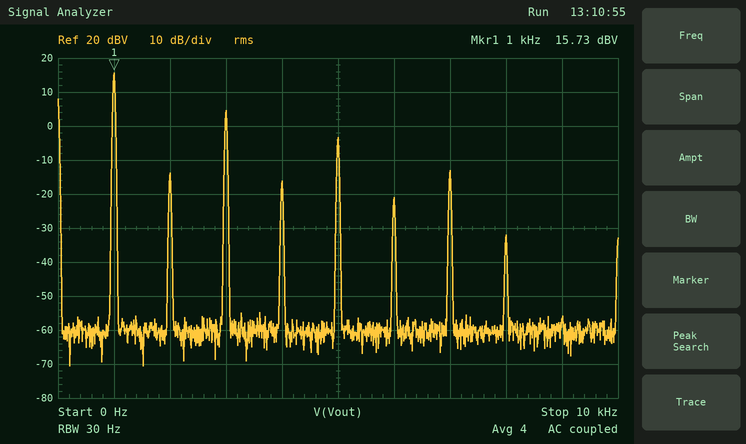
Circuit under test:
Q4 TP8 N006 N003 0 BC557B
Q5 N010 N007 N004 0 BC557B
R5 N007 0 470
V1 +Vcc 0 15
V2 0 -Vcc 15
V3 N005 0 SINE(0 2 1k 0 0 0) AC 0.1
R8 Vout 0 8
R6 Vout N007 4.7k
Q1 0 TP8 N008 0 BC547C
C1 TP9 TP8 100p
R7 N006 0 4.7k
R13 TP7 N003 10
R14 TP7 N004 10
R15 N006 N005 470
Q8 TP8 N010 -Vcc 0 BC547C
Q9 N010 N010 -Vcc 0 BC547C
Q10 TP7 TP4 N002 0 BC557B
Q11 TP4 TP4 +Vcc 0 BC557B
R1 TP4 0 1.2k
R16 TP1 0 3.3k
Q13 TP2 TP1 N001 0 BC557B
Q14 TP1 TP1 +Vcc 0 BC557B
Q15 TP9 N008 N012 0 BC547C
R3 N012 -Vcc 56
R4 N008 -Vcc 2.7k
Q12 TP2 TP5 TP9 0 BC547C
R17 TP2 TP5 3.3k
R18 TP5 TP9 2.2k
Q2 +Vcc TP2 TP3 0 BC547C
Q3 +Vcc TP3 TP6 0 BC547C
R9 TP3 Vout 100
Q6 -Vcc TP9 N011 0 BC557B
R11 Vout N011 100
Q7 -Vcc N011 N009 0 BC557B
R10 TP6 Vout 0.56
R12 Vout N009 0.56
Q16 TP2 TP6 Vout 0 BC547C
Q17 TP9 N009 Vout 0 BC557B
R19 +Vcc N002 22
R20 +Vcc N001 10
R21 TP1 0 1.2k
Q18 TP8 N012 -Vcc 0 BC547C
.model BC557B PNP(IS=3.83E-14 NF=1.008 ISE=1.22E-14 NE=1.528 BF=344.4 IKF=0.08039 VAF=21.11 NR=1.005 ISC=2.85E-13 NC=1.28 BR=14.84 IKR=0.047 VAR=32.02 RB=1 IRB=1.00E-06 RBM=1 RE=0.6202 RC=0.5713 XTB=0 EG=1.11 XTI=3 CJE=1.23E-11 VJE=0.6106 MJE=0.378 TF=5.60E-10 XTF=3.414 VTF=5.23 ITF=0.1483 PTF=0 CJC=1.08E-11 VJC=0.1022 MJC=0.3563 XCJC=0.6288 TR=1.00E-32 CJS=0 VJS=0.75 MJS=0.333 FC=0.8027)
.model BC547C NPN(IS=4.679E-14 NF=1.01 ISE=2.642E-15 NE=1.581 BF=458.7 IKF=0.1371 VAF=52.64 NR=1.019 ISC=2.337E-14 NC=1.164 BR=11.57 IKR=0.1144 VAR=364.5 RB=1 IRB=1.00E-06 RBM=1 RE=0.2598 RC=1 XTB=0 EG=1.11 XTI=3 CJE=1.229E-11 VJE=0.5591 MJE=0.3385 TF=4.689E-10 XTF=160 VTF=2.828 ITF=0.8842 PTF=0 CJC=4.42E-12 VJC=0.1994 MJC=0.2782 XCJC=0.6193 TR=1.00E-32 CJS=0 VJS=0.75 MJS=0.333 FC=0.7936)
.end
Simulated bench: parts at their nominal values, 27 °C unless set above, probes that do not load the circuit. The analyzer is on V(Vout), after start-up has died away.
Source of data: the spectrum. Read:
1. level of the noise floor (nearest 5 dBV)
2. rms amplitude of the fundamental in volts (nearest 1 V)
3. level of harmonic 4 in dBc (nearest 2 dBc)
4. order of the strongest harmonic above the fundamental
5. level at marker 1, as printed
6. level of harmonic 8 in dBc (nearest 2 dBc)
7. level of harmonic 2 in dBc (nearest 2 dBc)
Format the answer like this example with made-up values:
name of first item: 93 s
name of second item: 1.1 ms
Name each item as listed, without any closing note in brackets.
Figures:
level of the noise floor: -60 dBV
rms amplitude of the fundamental in volts: 6 V
level of harmonic 4 in dBc: -32 dBc
order of the strongest harmonic above the fundamental: 3
level at marker 1, as printed: 15.73 dBV
level of harmonic 8 in dBc: -48 dBc
level of harmonic 2 in dBc: -30 dBc
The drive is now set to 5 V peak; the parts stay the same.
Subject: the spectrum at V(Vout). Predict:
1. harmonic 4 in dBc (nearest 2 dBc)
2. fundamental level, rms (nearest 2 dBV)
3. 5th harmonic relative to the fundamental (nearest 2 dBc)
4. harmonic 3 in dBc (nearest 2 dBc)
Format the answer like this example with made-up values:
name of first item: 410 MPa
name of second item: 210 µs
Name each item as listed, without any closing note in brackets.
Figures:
harmonic 4 in dBc: -38 dBc
fundamental level, rms: 16 dBV
5th harmonic relative to the fundamental: -14 dBc
harmonic 3 in dBc: -10 dBc
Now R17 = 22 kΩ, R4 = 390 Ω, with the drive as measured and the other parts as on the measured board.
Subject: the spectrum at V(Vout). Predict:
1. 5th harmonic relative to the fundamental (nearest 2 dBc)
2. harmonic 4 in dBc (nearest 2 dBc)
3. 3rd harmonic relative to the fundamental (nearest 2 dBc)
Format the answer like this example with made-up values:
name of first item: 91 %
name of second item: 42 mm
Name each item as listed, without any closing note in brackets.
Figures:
5th harmonic relative to the fundamental: -24 dBc
harmonic 4 in dBc: -16 dBc
3rd harmonic relative to the fundamental: -12 dBc
